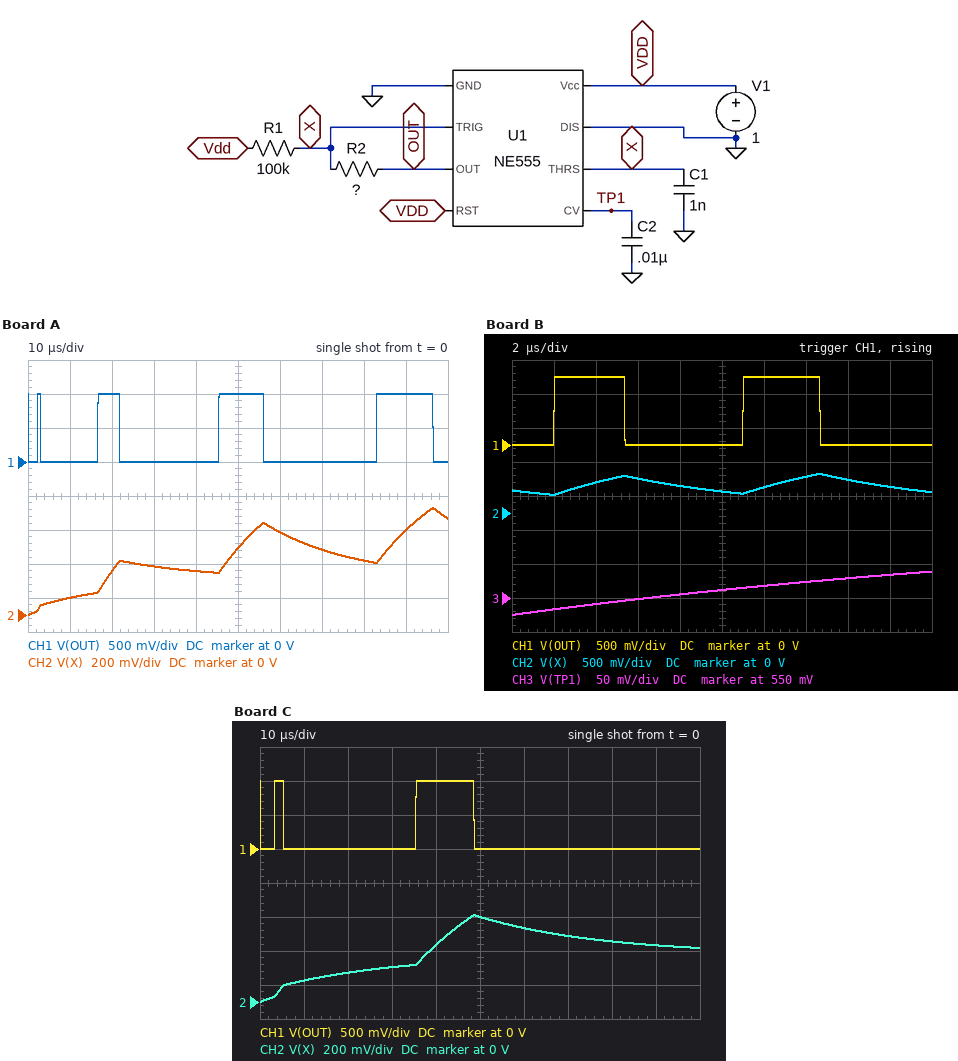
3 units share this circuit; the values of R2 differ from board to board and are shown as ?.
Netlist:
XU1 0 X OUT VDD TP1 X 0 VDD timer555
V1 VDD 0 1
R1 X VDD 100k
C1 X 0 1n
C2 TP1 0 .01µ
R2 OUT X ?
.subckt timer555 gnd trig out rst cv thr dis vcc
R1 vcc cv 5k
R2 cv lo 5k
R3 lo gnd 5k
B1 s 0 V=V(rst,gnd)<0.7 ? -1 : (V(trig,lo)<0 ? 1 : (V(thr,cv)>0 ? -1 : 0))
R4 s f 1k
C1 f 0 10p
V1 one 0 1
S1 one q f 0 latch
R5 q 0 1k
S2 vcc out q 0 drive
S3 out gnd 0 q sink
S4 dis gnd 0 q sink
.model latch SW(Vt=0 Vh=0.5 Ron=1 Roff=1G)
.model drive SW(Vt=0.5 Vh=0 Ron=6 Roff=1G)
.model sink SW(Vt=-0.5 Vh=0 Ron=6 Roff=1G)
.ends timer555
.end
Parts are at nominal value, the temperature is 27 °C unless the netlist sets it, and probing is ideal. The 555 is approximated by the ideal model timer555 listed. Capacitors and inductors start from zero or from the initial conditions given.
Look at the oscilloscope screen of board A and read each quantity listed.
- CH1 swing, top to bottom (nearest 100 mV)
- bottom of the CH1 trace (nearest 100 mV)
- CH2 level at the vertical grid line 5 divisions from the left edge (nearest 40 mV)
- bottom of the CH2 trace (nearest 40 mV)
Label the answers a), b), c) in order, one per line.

a) 1.0 V
b) 0 V
c) 400 mV
d) 0 V
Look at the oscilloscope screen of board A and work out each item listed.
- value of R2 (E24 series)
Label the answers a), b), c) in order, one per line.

a) 27 kΩ
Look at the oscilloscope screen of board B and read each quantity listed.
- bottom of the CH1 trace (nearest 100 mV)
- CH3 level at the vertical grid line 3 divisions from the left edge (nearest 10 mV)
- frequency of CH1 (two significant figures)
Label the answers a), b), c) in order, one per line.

a) 0 V
b) 550 mV
c) 110 kHz
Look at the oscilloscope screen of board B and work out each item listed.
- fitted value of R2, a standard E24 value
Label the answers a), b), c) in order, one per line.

a) 7.5 kΩ
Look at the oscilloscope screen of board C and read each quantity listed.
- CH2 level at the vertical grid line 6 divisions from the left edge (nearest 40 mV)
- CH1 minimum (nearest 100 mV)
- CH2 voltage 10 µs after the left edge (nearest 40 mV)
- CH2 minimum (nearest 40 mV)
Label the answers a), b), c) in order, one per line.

a) 440 mV
b) 0 V
c) 120 mV
d) 0 V
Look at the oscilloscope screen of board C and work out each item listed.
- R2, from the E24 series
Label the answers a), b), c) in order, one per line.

a) 39 kΩ
